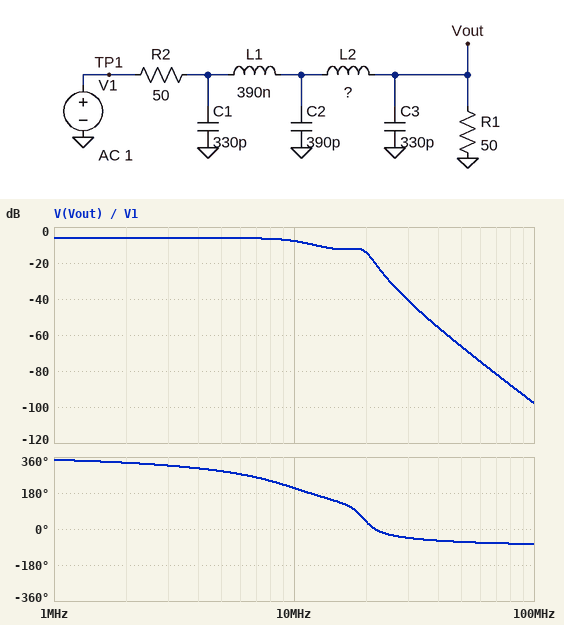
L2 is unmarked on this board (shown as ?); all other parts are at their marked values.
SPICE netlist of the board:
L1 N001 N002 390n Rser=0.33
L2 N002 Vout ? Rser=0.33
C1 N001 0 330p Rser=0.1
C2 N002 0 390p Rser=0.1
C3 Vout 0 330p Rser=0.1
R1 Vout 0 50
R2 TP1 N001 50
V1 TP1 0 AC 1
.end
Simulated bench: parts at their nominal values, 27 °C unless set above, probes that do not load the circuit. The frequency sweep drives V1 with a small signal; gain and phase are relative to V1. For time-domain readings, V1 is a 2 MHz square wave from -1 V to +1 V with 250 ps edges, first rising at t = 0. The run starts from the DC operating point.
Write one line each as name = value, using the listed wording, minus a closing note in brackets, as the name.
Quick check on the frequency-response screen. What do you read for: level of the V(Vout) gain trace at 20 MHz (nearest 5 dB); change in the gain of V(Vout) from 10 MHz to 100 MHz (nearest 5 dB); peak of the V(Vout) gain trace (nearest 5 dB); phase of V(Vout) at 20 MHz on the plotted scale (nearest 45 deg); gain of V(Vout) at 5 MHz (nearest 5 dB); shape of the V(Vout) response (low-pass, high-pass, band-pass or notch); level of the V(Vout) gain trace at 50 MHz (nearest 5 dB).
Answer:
level of the V(Vout) gain trace at 20 MHz = -15 dB
change in the gain of V(Vout) from 10 MHz to 100 MHz = -90 dB
peak of the V(Vout) gain trace = -5 dB
phase of V(Vout) at 20 MHz on the plotted scale = 45 deg
gain of V(Vout) at 5 MHz = -5 dB
shape of the V(Vout) response = low-pass
level of the V(Vout) gain trace at 50 MHz = -65 dB
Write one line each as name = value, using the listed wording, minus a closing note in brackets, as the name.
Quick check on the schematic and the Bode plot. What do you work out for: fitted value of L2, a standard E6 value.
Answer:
fitted value of L2, a standard E6 value = 1 µH
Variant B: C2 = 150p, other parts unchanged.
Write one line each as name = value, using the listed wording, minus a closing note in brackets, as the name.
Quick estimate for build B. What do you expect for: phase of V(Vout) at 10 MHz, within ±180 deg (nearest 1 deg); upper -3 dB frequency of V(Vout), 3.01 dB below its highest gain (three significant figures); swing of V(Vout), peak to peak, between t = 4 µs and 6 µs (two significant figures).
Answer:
phase of V(Vout) at 10 MHz, within ±180 deg = -139 deg
upper -3 dB frequency of V(Vout), 3.01 dB below its highest gain = 11.1 MHz
swing of V(Vout), peak to peak, between t = 4 µs and 6 µs = 1.2 V
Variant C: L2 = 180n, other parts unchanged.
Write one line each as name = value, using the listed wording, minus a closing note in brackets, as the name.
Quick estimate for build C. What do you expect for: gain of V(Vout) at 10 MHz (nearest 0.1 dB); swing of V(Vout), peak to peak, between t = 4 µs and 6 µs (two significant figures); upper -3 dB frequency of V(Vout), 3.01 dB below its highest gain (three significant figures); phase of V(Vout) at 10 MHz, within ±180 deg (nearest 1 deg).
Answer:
gain of V(Vout) at 10 MHz = -7.5 dB
swing of V(Vout), peak to peak, between t = 4 µs and 6 µs = 1.0 V
upper -3 dB frequency of V(Vout), 3.01 dB below its highest gain = 18.1 MHz
phase of V(Vout) at 10 MHz, within ±180 deg = -92 deg
